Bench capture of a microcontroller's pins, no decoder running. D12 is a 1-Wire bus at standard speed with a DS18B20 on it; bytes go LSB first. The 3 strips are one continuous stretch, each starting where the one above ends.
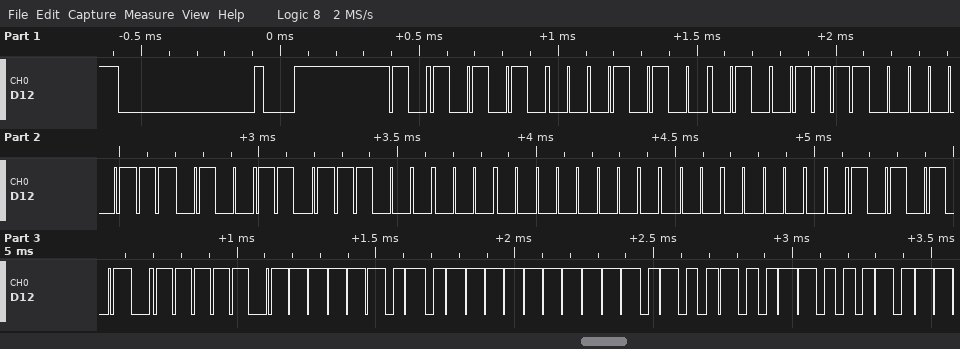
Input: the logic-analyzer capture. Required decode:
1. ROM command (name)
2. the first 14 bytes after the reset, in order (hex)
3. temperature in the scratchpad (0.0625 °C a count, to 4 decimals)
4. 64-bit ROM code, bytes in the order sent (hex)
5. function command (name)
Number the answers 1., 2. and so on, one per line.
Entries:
1. Match ROM
2. 55 28 F2 E0 B2 03 00 00 AA BE 5F FF 4B 46
3. -10.0625 °C
4. 28 F2 E0 B2 03 00 00 AA
5. Read Scratchpad
